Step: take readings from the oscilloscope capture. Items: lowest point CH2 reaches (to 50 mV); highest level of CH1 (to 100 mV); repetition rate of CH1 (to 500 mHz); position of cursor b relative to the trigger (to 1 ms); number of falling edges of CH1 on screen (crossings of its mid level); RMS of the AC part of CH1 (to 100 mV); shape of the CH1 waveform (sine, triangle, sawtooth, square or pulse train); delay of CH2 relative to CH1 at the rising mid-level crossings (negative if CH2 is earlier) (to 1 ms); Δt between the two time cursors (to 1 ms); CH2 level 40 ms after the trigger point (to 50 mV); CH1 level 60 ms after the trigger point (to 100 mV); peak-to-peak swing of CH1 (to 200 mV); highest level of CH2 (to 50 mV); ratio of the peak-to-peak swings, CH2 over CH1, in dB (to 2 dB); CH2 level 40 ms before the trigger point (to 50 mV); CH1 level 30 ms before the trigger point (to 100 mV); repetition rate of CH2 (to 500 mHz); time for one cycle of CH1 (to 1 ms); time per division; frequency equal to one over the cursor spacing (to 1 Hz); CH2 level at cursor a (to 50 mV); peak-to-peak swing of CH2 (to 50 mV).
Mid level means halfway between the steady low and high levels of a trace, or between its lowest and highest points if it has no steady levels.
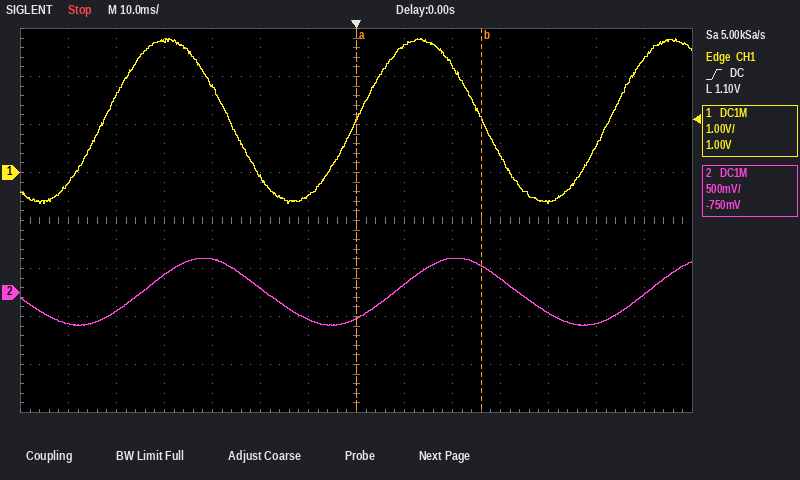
-350 mV
2.8 V
19.0 Hz
+26 ms
2
1.2 V
sine
+8 ms
26 ms
-200 mV
2.4 V
3.4 V
350 mV
-14 dB
200 mV
1.8 V
19.0 Hz
53 ms
10 ms
38 Hz
-250 mV
700 mV
